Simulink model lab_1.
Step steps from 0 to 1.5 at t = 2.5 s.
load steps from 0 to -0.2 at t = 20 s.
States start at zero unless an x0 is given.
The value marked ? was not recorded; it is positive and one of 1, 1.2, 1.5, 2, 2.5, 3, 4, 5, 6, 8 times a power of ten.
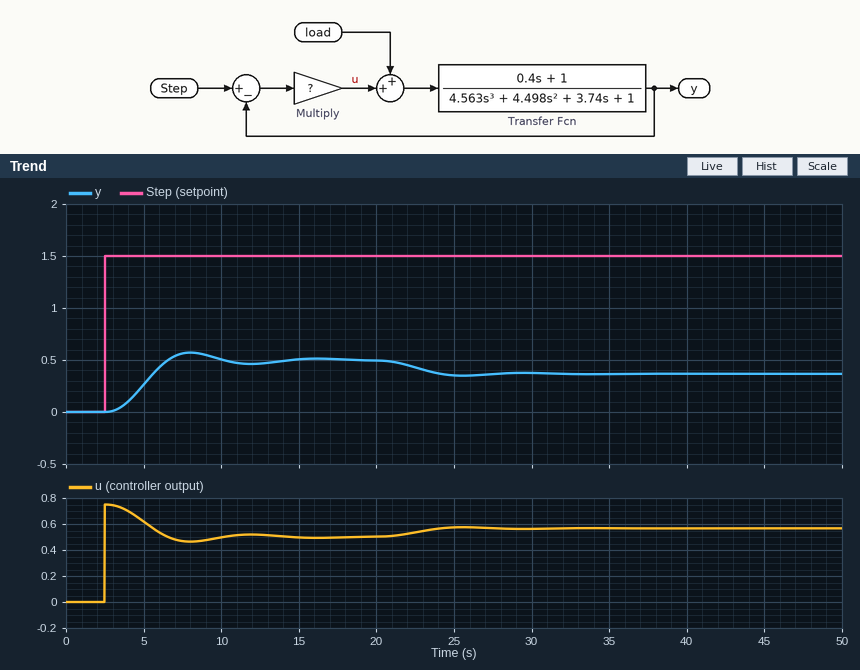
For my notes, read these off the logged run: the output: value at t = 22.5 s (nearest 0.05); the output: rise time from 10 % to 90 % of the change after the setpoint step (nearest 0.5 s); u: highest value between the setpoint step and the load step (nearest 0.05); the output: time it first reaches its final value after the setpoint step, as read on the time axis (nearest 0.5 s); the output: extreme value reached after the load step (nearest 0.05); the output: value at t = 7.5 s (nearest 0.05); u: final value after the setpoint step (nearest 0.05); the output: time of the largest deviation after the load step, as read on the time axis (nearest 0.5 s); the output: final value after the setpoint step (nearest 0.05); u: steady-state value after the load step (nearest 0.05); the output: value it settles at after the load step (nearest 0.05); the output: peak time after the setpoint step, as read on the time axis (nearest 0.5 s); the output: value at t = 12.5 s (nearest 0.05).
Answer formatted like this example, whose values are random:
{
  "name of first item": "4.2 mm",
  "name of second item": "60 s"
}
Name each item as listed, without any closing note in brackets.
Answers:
{
  "the output: value at t = 22.5 s": "0.45",
  "the output: rise time from 10 % to 90 % of the change after the setpoint step": "2.5 s",
  "u: highest value between the setpoint step and the load step": "0.75",
  "the output: time it first reaches its final value after the setpoint step, as read on the time axis": "6.5 s",
  "the output: extreme value reached after the load step": "0.35",
  "the output: value at t = 7.5 s": "0.55",
  "u: final value after the setpoint step": "0.50",
  "the output: time of the largest deviation after the load step, as read on the time axis": "25.5 s",
  "the output: final value after the setpoint step": "0.50",
  "u: steady-state value after the load step": "0.55",
  "the output: value it settles at after the load step": "0.35",
  "the output: peak time after the setpoint step, as read on the time axis": "8.0 s",
  "the output: value at t = 12.5 s": "0.45"
}
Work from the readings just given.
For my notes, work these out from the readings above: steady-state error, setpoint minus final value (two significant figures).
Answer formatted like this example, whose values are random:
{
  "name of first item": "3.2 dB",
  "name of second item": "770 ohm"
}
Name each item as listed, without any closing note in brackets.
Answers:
{
  "steady-state error, setpoint minus final value": "1.0"
}
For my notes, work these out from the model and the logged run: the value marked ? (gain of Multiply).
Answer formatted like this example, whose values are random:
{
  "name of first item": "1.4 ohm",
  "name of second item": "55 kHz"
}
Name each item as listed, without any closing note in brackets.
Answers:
{
  "the value marked ?": "0.5"
}
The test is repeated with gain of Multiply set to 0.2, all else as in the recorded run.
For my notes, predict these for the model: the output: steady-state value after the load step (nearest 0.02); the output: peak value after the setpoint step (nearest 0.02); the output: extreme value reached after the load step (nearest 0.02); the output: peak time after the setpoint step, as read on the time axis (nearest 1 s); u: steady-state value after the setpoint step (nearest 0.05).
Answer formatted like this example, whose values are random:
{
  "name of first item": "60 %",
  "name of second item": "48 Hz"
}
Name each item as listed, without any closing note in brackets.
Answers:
{
  "the output: steady-state value after the load step": "0.08",
  "the output: peak value after the setpoint step": "0.26",
  "the output: extreme value reached after the load step": "0.08",
  "the output: peak time after the setpoint step, as read on the time axis": "9 s",
  "u: steady-state value after the setpoint step": "0.25"
}
